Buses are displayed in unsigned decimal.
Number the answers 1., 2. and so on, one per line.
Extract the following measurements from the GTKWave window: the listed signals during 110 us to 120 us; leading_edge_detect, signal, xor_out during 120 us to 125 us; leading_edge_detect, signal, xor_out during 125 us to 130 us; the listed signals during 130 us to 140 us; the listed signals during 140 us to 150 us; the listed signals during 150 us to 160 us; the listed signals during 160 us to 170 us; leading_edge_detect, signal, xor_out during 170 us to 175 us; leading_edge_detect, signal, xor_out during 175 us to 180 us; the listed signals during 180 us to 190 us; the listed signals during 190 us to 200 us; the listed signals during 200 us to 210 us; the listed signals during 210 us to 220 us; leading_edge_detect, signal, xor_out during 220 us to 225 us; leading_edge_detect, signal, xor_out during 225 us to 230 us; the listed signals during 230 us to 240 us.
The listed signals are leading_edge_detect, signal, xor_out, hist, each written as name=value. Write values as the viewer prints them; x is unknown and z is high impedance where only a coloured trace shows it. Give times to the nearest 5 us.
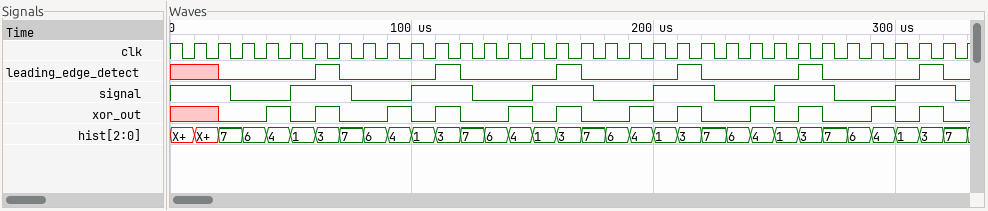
1. leading_edge_detect=1, signal=1, xor_out=1, hist=3
2. leading_edge_detect=0, signal=1, xor_out=0
3. leading_edge_detect=0, signal=0, xor_out=0
4. leading_edge_detect=0, signal=0, xor_out=0, hist=6
5. leading_edge_detect=0, signal=0, xor_out=1, hist=4
6. leading_edge_detect=0, signal=1, xor_out=0, hist=1
7. leading_edge_detect=1, signal=1, xor_out=1, hist=3
8. leading_edge_detect=0, signal=1, xor_out=0
9. leading_edge_detect=0, signal=0, xor_out=0
10. leading_edge_detect=0, signal=0, xor_out=0, hist=6
11. leading_edge_detect=0, signal=0, xor_out=1, hist=4
12. leading_edge_detect=0, signal=1, xor_out=0, hist=1
13. leading_edge_detect=1, signal=1, xor_out=1, hist=3
14. leading_edge_detect=0, signal=1, xor_out=0
15. leading_edge_detect=0, signal=0, xor_out=0
16. leading_edge_detect=0, signal=0, xor_out=0, hist=6
